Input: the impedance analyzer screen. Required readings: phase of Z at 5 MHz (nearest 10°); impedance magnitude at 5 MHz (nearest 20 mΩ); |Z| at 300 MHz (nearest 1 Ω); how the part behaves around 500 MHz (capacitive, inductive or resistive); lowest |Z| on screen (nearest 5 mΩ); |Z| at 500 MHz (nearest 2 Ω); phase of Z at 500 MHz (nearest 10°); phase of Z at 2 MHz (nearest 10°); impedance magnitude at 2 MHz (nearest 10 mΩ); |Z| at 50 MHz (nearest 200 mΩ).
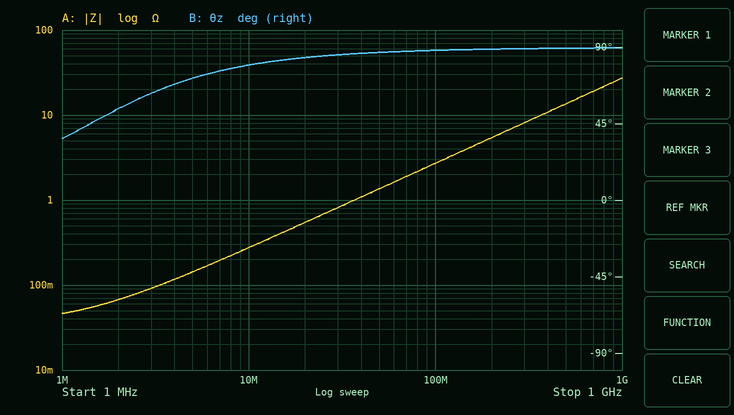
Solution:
70°
140 mΩ
8 Ω
inductive
45 mΩ
14 Ω
90°
50°
70 mΩ
1.4 Ω
